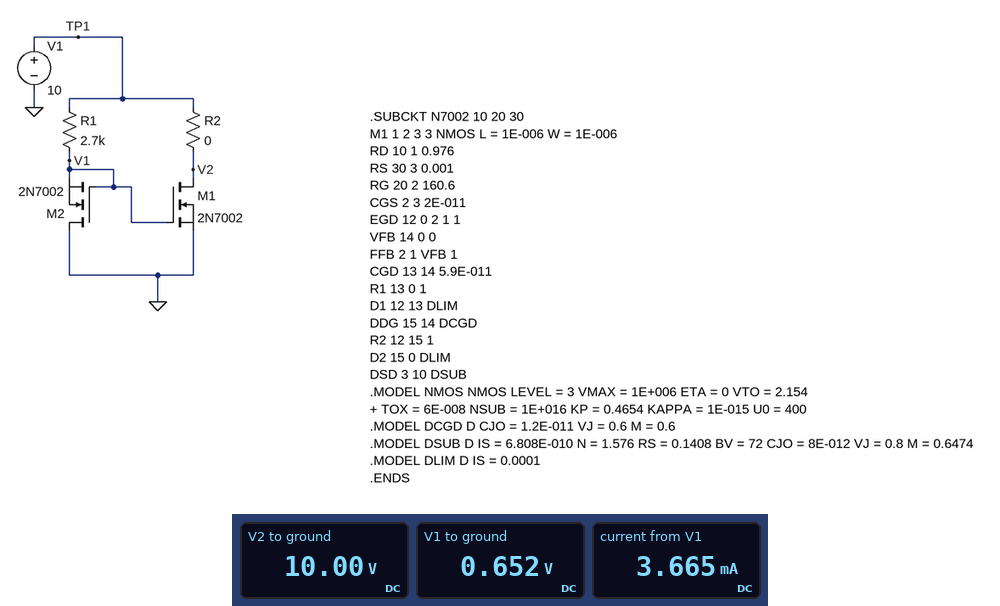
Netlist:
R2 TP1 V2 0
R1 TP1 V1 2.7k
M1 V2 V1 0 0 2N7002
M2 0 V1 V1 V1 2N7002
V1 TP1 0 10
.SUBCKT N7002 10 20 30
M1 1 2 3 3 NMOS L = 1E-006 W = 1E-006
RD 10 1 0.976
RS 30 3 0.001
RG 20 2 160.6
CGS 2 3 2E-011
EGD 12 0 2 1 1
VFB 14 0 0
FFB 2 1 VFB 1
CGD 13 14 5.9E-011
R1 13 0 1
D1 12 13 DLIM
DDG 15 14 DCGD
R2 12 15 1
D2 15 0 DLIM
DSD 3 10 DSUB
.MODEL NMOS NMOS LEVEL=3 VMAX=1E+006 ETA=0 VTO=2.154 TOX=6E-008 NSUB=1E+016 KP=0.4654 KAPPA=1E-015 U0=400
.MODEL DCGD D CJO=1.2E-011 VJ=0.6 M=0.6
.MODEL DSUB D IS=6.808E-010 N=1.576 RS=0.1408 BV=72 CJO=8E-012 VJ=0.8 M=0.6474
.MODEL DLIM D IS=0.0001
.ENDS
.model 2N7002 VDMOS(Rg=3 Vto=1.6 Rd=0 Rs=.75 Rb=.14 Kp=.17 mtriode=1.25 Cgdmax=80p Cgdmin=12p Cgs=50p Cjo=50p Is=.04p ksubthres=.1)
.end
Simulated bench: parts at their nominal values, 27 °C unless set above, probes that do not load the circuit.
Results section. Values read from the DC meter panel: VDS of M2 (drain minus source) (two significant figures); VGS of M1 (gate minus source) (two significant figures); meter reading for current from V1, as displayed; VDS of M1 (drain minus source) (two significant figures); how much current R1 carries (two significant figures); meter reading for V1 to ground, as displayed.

-650 mV
650 mV
3.665 mA
10 V
3.5 mA
0.652 V
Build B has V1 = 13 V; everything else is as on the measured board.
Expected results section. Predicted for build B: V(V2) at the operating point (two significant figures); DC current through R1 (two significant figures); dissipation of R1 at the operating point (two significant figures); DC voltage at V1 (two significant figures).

13 V
4.6 mA
56 mW
660 mV
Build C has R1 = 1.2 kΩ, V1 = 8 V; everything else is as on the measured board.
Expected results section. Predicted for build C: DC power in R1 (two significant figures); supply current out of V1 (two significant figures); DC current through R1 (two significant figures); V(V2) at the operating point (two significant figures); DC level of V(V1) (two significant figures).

45 mW
6.3 mA
6.1 mA
8.0 V
670 mV
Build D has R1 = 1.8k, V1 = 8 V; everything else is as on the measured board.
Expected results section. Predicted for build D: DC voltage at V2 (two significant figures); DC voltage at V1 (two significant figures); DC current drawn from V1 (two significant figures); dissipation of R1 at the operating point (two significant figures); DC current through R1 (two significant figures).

8.0 V
660 mV
4.5 mA
30 mW
4.1 mA
